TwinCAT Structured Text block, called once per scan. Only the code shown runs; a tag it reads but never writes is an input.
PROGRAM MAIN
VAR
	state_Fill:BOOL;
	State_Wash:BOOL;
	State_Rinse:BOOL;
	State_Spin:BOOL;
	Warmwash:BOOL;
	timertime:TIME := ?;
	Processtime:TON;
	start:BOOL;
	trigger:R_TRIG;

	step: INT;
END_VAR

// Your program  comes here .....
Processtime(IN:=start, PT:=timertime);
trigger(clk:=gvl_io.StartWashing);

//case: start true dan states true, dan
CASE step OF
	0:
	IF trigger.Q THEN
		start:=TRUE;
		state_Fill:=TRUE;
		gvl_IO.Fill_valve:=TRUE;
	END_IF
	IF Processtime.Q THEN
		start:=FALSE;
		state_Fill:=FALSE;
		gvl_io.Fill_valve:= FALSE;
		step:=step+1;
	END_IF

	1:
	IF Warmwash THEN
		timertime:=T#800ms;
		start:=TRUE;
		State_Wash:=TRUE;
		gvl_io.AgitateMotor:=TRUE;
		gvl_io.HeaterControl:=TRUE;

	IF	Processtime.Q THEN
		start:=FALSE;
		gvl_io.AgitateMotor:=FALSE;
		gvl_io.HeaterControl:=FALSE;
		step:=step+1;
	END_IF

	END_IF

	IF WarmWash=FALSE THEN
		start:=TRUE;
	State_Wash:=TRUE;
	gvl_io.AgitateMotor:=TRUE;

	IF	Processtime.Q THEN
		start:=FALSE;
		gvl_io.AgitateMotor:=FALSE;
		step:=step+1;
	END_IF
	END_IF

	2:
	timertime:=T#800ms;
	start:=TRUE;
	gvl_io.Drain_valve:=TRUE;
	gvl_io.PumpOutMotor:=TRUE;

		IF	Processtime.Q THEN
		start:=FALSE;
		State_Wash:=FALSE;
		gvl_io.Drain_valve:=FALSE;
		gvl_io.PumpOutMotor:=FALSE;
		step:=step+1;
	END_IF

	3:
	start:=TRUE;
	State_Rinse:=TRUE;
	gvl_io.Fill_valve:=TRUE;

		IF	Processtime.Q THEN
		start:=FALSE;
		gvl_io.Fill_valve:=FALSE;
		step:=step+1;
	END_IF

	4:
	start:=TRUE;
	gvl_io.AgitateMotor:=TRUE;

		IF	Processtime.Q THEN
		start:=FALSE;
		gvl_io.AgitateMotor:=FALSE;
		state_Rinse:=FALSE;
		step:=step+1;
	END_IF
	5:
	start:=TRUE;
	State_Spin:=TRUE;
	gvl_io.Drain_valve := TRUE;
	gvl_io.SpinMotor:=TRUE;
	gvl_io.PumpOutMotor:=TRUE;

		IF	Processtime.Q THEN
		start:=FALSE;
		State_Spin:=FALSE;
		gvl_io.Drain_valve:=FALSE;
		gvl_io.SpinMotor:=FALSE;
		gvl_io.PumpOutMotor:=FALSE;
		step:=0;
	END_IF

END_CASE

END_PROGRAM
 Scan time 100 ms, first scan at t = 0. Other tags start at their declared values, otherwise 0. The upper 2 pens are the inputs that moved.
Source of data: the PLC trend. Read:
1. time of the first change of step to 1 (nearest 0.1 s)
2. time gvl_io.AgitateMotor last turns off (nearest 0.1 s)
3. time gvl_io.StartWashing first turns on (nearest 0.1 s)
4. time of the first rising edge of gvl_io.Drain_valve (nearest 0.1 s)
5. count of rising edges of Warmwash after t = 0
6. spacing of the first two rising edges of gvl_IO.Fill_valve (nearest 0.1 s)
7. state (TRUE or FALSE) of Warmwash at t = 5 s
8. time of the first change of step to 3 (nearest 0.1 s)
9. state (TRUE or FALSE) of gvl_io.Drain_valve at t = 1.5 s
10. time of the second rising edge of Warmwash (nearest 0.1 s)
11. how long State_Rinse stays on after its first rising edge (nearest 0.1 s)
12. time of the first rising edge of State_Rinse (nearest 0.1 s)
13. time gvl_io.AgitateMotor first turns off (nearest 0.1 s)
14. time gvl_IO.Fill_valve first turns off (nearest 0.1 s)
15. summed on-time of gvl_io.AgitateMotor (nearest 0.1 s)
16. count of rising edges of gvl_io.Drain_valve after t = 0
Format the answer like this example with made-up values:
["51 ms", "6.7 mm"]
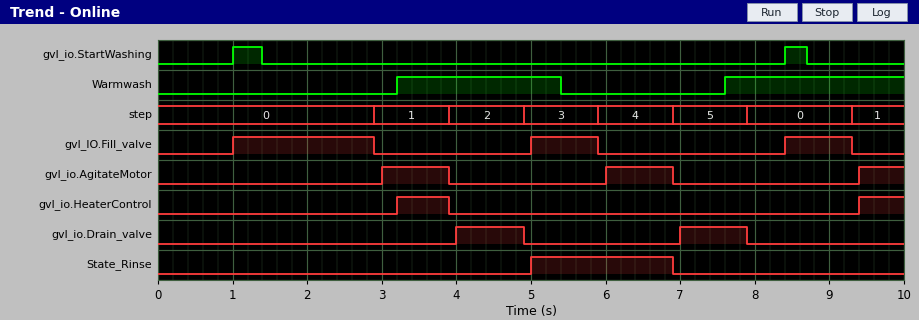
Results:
["2.9 s", "6.9 s", "1.0 s", "4.0 s", "2", "4.0 s", "TRUE", "4.9 s", "FALSE", "7.6 s", "1.9 s", "5.0 s", "3.9 s", "2.9 s", "2.4 s", "2"]
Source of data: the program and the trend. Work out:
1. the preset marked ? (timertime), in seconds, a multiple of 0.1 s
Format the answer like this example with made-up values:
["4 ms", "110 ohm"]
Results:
["1.8 s"]
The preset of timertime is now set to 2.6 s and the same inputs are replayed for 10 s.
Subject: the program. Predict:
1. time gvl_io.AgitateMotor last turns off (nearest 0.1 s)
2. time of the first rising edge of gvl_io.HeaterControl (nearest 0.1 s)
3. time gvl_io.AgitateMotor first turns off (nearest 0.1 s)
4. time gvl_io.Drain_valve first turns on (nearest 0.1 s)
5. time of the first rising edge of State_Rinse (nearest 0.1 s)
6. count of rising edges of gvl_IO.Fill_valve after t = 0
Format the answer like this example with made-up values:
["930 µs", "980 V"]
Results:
["7.7 s", "3.8 s", "4.7 s", "4.8 s", "5.8 s", "2"]
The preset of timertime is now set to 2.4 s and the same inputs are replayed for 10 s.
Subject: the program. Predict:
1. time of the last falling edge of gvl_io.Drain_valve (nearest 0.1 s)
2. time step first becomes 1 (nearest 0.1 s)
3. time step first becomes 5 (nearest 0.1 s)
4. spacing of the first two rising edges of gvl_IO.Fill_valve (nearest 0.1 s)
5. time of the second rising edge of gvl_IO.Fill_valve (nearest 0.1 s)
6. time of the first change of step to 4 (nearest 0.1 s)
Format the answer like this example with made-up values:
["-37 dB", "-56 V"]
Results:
["8.5 s", "3.5 s", "7.5 s", "4.6 s", "5.6 s", "6.5 s"]
